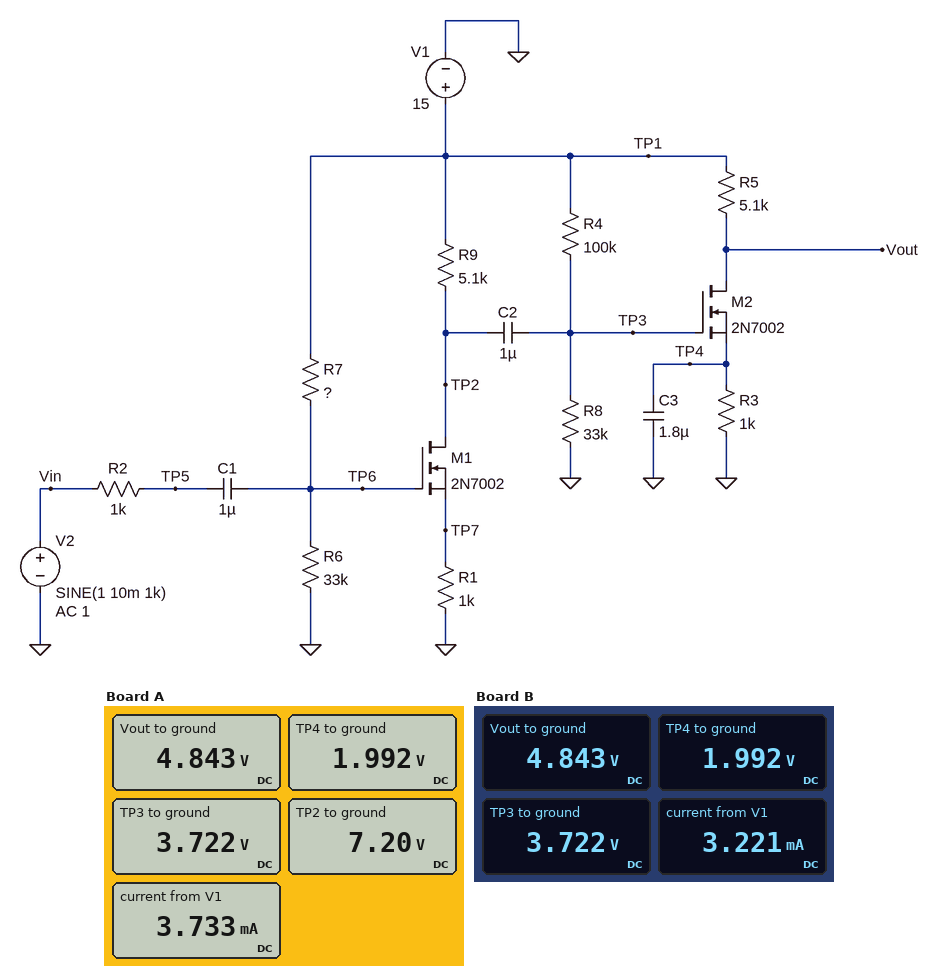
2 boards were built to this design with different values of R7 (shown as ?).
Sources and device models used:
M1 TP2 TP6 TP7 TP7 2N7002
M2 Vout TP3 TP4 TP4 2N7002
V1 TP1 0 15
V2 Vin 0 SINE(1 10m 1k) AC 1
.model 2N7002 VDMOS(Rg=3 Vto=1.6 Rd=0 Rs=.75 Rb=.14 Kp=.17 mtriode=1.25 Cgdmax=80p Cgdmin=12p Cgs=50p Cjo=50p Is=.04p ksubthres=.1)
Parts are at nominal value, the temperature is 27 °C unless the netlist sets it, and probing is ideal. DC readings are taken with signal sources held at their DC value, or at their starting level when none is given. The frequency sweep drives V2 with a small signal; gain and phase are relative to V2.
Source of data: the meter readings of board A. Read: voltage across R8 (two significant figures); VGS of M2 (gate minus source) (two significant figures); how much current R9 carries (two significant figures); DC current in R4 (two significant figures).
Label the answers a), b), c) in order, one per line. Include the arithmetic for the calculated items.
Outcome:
a) 3.722 V = 3.7 V
b) 3.722 V - 1.992 V = 1.7 V
c) (15 V - 7.2 V) / 5.1 kΩ = 1.5 mA
d) (15 V - 3.722 V) / 100 kΩ = 110 µA
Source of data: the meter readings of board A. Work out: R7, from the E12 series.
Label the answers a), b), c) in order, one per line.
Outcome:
a) 120 kΩ
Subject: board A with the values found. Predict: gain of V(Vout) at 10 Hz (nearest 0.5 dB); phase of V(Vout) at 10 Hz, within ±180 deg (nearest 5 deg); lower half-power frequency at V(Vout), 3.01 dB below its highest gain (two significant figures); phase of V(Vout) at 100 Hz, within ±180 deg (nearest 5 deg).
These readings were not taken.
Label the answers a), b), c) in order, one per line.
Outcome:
a) 23.0 dB
b) 65 deg
c) 1.6 kHz
d) 50 deg
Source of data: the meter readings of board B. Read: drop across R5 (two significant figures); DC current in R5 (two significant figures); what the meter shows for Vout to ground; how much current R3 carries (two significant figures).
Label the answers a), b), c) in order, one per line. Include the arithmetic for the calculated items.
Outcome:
a) 15 V - 4.843 V = 10 V
b) (15 V - 4.843 V) / 5.1 kΩ = 2.0 mA
c) 4.843 V
d) (1.992 V) / 1 kΩ = 2.0 mA
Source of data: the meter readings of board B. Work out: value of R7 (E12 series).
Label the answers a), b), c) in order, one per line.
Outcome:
a) 150 kΩ
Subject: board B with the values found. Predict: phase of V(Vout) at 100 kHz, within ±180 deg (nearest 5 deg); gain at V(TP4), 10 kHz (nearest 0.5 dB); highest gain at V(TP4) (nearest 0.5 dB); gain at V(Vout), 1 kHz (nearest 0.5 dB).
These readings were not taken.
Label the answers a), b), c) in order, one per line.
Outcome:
a) -85 deg
b) -5.5 dB
c) 11.0 dB
d) 45.5 dB
